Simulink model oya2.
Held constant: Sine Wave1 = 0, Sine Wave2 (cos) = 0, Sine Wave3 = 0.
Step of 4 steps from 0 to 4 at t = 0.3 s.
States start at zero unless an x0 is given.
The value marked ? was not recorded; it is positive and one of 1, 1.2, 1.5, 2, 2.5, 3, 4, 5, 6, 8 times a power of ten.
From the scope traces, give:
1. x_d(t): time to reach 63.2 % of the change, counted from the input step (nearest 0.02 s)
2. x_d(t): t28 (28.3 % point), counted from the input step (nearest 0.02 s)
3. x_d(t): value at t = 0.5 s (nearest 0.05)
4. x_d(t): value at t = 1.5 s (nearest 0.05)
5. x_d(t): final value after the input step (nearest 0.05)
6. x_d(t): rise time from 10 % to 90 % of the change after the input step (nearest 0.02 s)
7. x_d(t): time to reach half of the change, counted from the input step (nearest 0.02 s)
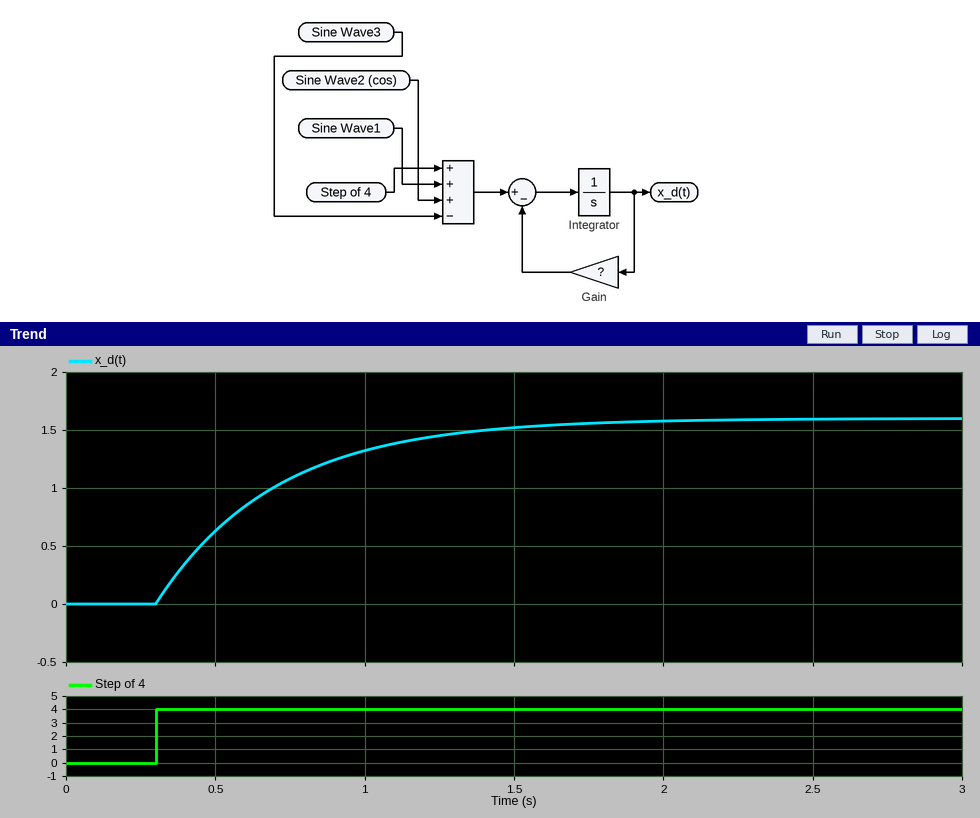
0.40 s
0.14 s
0.65
1.50
1.60
0.88 s
0.28 s
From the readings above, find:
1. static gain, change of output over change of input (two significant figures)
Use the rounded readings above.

0.40
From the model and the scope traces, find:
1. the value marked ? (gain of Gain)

2.5
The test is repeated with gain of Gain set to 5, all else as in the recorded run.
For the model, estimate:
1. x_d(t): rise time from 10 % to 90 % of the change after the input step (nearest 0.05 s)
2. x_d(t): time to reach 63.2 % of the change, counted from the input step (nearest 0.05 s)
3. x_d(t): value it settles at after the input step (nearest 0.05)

0.45 s
0.20 s
0.80
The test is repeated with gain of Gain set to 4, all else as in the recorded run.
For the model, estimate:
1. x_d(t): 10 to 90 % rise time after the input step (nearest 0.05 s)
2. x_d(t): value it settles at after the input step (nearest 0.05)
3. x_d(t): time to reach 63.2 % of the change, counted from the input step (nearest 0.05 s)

0.55 s
1.00
0.25 s
